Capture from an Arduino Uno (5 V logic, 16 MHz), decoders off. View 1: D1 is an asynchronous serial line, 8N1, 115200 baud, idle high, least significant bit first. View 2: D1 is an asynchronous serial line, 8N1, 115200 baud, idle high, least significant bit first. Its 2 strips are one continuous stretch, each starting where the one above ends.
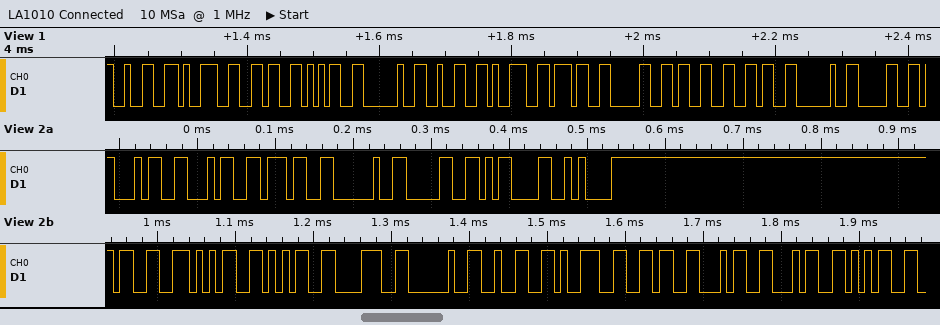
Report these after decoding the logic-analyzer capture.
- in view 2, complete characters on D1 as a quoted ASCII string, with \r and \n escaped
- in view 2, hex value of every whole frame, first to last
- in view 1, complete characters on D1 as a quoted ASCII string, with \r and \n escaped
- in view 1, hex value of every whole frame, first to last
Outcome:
"447 0\r\n3558 296445"
34 34 37 20 30 0D 0A 33 35 35 38 20 32 39 36 34 34 35
"2965 297036 0"
32 39 36 35 20 32 39 37 30 33 36 20 30
